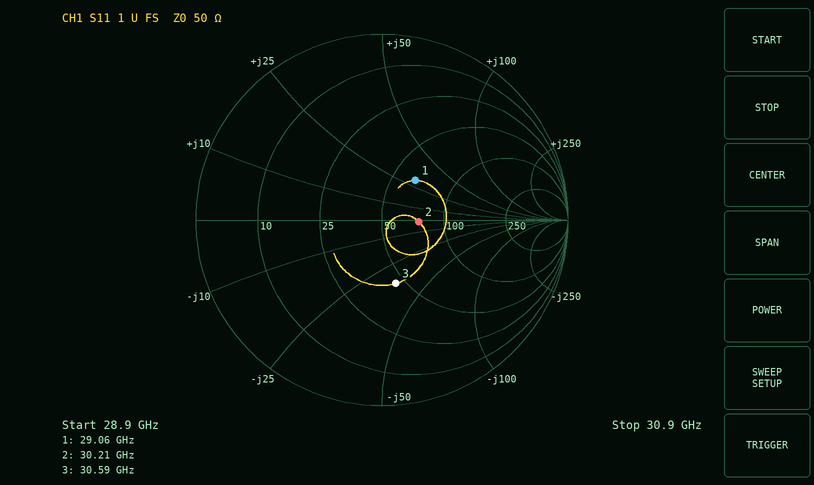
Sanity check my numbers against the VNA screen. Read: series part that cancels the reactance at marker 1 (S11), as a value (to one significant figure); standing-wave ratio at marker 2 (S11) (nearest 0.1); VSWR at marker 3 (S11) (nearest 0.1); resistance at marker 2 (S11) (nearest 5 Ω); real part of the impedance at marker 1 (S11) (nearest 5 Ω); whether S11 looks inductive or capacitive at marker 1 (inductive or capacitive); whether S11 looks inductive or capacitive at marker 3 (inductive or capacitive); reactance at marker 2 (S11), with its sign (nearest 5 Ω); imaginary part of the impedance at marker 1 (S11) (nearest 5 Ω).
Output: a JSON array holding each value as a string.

["200 fF", "1.5", "2.1", "75 Ω", "65 Ω", "inductive", "capacitive", "0 Ω", "+30 Ω"]
